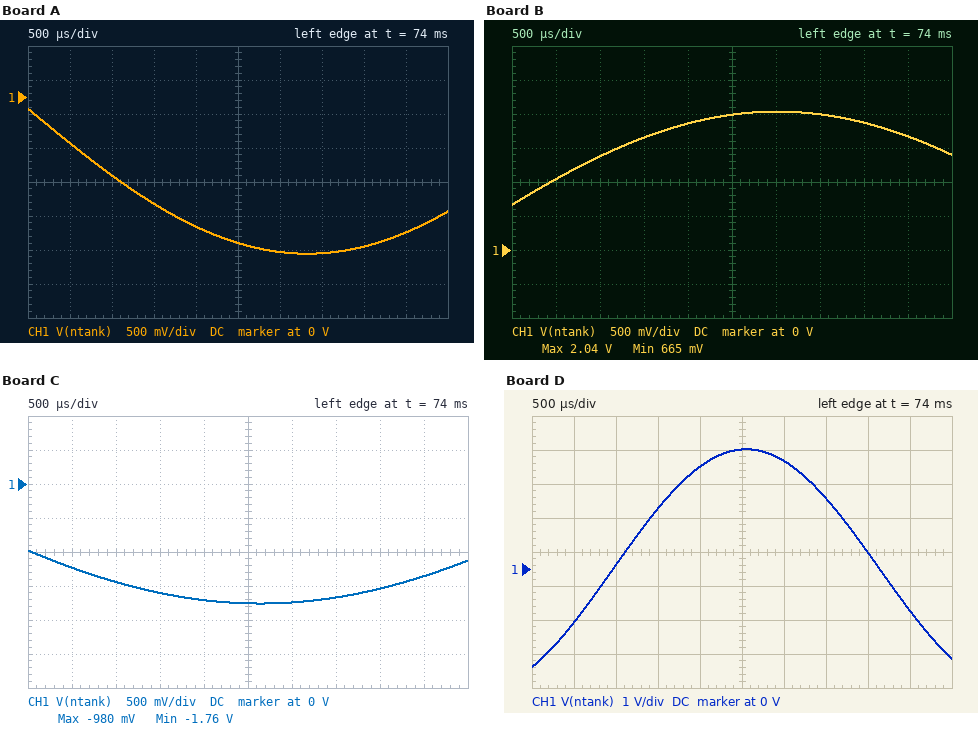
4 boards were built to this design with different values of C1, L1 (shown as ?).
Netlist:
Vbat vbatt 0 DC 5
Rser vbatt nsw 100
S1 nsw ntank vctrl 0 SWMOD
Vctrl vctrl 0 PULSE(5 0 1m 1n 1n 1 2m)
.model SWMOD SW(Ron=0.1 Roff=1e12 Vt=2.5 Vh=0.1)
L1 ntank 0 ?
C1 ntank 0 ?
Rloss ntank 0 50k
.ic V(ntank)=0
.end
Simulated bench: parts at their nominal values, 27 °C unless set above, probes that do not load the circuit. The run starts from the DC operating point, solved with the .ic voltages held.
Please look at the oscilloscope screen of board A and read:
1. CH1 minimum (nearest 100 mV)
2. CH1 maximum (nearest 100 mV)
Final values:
-2.3 V
-200 mV
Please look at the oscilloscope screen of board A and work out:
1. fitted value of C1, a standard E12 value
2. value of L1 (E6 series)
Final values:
15 µF
330 mH
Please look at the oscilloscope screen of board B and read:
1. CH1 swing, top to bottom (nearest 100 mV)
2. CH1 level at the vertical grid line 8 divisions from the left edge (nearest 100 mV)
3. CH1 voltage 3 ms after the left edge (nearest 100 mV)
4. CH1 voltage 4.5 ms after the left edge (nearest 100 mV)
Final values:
1.4 V
1.9 V
2.0 V
1.7 V
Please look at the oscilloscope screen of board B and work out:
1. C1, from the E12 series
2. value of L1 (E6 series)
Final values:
18 µF
330 mH
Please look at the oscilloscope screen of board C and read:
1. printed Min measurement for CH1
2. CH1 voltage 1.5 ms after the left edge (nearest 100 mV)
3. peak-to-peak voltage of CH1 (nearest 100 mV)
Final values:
-1.76 V
-1.6 V
800 mV
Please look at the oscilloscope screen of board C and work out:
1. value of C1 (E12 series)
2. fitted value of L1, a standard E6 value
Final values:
22 µF
330 mH
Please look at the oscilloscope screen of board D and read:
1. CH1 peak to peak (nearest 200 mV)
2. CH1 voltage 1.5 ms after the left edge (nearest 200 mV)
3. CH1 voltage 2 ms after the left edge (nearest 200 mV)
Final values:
6.4 V
1.8 V
3.0 V
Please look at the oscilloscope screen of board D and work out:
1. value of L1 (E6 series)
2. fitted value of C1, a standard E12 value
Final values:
150 mH
6.8 µF
